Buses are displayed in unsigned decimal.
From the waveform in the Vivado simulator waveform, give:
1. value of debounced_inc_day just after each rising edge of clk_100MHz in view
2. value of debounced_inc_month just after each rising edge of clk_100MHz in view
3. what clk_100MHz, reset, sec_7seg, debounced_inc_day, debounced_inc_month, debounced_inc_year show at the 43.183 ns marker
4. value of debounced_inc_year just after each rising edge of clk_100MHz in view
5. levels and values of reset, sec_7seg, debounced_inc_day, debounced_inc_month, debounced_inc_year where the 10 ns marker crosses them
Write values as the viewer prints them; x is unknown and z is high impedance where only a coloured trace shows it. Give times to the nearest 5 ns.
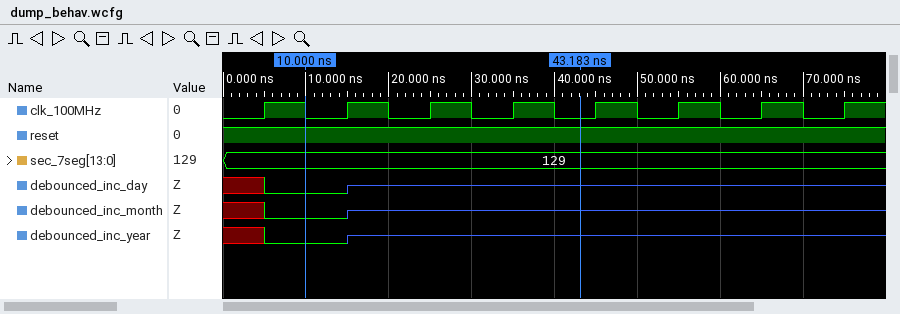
0 z z z z z z z
0 z z z z z z z
clk_100MHz=0, reset=1, sec_7seg=129, debounced_inc_day=z, debounced_inc_month=z, debounced_inc_year=z
0 z z z z z z z
reset=1, sec_7seg=129, debounced_inc_day=0, debounced_inc_month=0, debounced_inc_year=0
